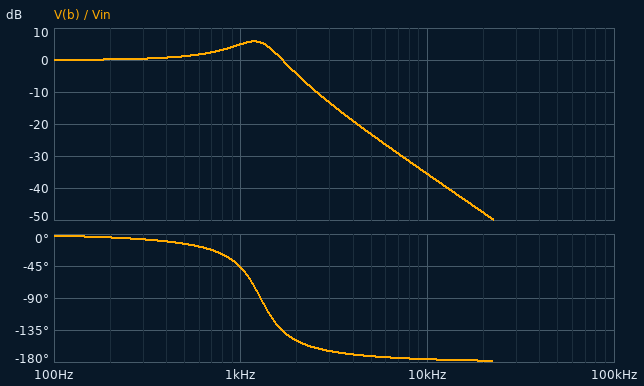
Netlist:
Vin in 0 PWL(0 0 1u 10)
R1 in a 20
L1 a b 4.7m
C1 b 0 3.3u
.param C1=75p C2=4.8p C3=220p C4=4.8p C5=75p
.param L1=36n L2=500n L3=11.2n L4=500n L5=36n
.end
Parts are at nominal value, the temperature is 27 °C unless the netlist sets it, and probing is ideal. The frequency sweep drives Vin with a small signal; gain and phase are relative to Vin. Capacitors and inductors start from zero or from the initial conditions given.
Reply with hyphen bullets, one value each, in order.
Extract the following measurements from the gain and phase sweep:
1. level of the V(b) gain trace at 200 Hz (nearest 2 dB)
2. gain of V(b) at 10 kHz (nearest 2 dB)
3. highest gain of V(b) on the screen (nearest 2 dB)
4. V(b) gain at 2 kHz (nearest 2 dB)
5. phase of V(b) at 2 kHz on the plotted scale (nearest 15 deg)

- 0 dB
- -36 dB
- 6 dB
- -4 dB
- -150 deg
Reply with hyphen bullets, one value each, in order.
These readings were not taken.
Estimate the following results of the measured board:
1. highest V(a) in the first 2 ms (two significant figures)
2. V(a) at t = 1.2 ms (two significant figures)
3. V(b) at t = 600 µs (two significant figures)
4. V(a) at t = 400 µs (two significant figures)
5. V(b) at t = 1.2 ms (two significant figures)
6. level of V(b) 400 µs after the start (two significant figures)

- 12 V
- 9.9 V
- 11 V
- 9.9 V
- 11 V
- 14 V
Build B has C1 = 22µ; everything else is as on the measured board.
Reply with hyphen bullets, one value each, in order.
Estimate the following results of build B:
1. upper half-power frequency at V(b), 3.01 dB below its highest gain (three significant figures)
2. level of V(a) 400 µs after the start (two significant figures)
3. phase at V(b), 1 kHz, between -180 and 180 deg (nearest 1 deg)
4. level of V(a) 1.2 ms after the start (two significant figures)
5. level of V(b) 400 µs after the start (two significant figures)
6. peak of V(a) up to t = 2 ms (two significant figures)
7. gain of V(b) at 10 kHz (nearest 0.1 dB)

- 510 Hz
- 3.7 V
- -138 deg
- 9.4 V
- 4.2 V
- 10 V
- -52.2 dB
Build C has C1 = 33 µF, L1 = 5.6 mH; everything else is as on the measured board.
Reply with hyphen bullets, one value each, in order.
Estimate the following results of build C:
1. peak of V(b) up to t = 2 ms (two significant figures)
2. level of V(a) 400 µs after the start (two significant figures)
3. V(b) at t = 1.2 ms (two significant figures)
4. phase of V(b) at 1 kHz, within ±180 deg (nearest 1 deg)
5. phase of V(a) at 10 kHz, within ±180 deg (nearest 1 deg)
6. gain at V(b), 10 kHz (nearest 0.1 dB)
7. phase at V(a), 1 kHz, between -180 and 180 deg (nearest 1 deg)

- 10 V
- 3.4 V
- 8.9 V
- -147 deg
- 3 deg
- -57.3 dB
- 33 deg
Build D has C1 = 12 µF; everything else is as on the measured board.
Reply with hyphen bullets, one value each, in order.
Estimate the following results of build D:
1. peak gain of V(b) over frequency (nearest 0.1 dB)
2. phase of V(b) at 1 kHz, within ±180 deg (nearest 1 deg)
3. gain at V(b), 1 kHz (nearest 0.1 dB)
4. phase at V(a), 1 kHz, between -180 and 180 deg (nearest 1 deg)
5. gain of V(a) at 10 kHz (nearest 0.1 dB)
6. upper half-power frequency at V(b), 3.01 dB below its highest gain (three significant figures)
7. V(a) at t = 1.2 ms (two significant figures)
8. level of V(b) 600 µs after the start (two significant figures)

- 1.2 dB
- -129 deg
- -5.8 dB
- 51 deg
- 0 dB
- 782 Hz
- 11 V
- 10 V
